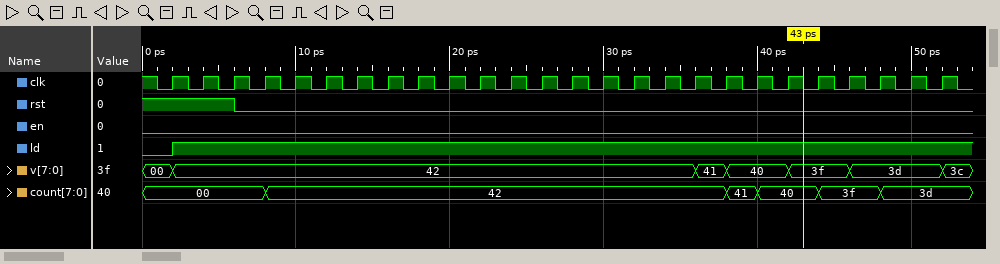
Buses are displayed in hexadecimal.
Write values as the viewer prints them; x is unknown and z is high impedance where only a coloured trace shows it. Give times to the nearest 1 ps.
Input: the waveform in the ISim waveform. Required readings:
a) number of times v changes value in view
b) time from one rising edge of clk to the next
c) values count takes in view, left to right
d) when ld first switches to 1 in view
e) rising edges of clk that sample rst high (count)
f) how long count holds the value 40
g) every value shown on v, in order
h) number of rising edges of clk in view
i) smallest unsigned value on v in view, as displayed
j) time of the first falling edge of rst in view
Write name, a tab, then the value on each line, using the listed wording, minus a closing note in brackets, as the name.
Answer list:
number of times v changes value in view	6
time from one rising edge of clk to the next	2 ps
values count takes in view, left to right	00, 42, 41, 40, 3f, 3d
when ld first switches to 1 in view	2 ps
rising edges of clk that sample rst high	3
how long count holds the value 40	4 ps
every value shown on v, in order	00, 42, 41, 40, 3f, 3d, 3c
number of rising edges of clk in view	26
smallest unsigned value on v in view, as displayed	00
time of the first falling edge of rst in view	6 ps
